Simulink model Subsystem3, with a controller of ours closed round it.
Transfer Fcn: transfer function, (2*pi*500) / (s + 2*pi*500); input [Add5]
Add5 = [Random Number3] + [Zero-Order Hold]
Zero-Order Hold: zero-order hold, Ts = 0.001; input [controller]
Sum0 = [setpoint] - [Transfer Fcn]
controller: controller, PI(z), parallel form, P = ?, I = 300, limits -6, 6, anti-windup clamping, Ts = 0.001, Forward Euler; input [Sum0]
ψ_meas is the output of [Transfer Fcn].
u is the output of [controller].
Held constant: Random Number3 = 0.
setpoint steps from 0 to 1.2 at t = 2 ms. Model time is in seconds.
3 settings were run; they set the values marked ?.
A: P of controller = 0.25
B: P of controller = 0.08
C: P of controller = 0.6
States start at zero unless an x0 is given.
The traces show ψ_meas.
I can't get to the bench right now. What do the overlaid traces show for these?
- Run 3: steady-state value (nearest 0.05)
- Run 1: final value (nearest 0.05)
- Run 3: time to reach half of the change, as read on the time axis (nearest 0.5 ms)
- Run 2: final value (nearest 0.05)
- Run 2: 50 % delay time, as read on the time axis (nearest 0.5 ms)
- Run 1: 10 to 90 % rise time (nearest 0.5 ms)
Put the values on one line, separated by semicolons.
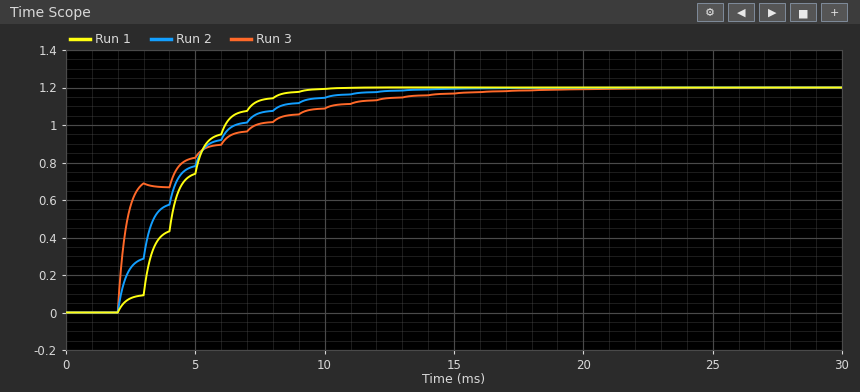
1.20; 1.20; 2.5 ms; 1.20; 4.0 ms; 4.0 ms
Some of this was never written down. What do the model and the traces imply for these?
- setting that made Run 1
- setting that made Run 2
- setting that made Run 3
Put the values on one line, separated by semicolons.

B; A; C
